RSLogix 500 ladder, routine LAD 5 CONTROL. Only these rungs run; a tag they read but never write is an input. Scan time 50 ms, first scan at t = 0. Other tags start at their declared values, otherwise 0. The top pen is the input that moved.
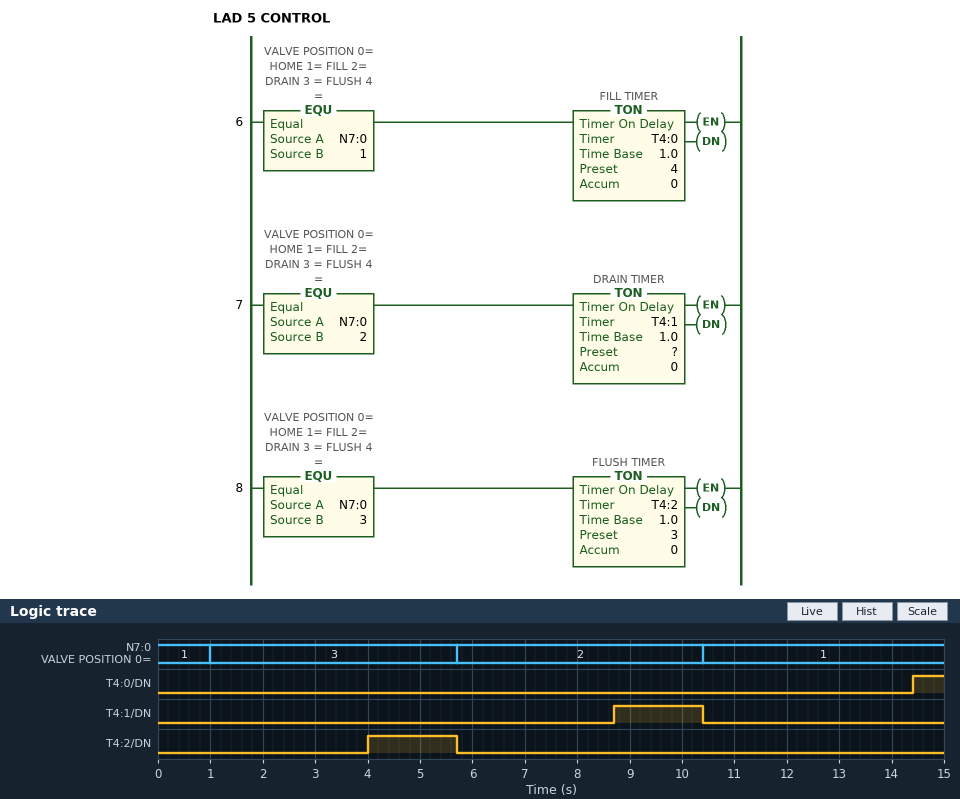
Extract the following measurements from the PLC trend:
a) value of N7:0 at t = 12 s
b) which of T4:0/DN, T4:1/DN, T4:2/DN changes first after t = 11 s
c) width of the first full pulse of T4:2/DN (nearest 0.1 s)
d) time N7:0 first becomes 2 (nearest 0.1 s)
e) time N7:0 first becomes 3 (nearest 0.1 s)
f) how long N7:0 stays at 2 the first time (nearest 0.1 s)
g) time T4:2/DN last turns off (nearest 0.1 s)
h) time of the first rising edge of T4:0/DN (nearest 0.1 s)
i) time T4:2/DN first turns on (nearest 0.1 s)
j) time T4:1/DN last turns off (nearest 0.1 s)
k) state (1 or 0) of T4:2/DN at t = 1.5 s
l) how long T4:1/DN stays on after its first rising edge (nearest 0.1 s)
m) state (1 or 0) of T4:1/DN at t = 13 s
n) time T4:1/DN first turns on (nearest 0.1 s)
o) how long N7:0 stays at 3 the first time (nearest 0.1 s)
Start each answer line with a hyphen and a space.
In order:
- 1
- T4:0/DN
- 1.7 s
- 5.7 s
- 1.0 s
- 4.7 s
- 5.7 s
- 14.4 s
- 4.0 s
- 10.4 s
- 0
- 1.7 s
- 0
- 8.7 s
- 4.7 s
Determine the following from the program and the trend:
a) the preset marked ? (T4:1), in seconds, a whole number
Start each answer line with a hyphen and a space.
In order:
- 3 s
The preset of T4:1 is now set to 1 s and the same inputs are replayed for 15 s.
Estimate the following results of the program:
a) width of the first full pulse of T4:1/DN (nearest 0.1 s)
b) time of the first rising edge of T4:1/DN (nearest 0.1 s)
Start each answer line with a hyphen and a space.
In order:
- 3.7 s
- 6.7 s
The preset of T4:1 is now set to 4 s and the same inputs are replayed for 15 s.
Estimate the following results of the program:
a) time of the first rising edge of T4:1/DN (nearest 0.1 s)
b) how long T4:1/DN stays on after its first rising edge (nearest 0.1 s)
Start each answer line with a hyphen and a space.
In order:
- 9.7 s
- 0.7 s
